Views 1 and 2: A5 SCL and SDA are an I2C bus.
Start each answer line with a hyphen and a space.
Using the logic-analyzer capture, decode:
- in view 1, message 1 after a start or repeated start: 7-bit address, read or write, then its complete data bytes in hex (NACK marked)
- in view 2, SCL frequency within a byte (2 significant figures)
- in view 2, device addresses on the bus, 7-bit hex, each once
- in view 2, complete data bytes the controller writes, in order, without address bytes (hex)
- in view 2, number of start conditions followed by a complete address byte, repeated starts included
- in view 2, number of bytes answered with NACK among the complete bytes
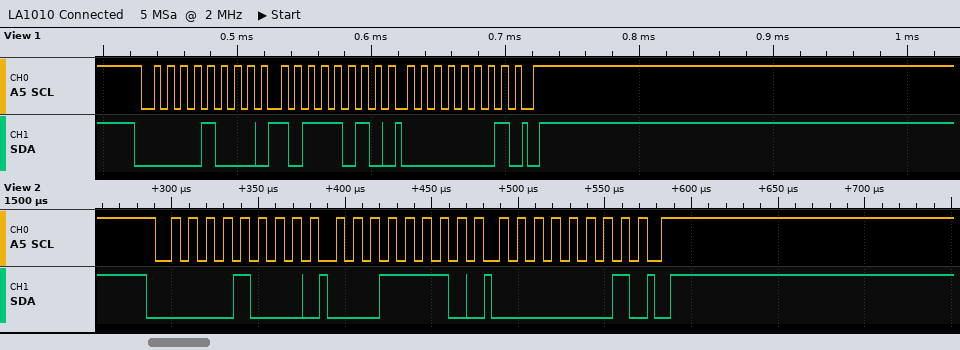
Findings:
- 0x04 write: BA 01
- 100 kHz
- 0x04
- 1E 01
- 1
- 0
